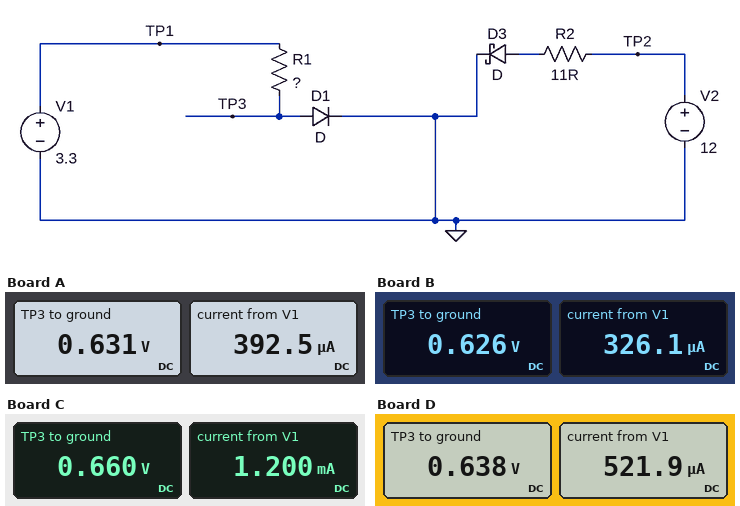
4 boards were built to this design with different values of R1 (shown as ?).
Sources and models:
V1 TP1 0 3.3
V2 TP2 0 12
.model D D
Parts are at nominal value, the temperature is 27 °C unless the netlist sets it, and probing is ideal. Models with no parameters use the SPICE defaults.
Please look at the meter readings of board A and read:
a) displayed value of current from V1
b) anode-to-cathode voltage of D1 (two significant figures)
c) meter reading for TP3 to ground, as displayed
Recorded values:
392.5 µA
630 mV
0.631 V
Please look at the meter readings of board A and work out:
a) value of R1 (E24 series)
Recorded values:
6.8 kΩ
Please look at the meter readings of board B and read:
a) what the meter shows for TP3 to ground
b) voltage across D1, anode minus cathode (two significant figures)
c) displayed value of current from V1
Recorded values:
0.626 V
630 mV
326.1 µA
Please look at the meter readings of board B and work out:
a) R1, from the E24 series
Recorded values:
8.2 kΩ
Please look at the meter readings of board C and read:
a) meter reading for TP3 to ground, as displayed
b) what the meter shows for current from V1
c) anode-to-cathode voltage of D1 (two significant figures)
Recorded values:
0.660 V
1.200 mA
660 mV
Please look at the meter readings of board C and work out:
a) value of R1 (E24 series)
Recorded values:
2.2 kΩ
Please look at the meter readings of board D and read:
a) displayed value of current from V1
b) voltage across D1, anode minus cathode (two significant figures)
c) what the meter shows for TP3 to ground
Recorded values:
521.9 µA
640 mV
0.638 V
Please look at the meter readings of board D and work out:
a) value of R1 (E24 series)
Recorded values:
5.1 kΩ
